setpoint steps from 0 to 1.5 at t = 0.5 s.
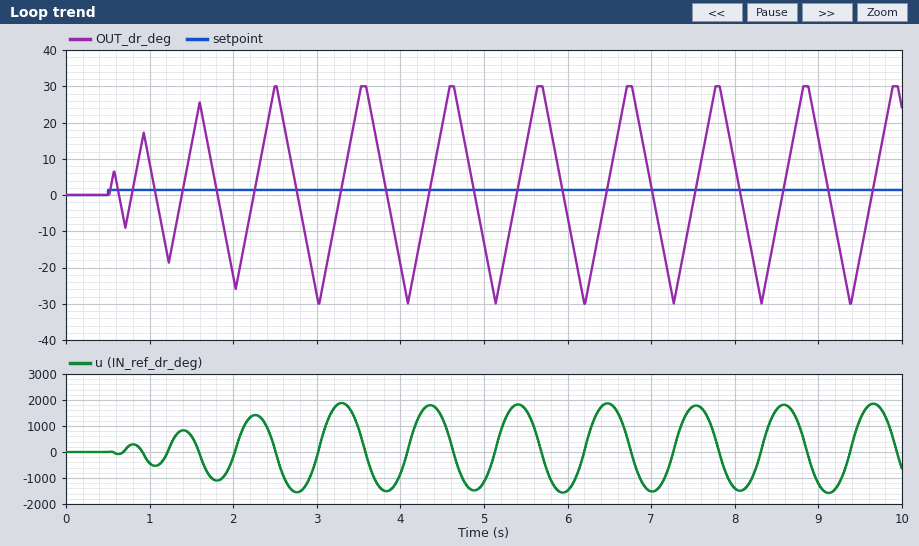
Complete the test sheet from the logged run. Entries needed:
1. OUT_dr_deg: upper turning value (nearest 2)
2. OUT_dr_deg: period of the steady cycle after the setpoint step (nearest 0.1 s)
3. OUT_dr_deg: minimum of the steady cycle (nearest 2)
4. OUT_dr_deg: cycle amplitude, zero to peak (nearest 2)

30
1.1 s
-30
30
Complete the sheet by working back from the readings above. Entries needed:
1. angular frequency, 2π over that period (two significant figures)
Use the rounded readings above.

5.7 rad/s
